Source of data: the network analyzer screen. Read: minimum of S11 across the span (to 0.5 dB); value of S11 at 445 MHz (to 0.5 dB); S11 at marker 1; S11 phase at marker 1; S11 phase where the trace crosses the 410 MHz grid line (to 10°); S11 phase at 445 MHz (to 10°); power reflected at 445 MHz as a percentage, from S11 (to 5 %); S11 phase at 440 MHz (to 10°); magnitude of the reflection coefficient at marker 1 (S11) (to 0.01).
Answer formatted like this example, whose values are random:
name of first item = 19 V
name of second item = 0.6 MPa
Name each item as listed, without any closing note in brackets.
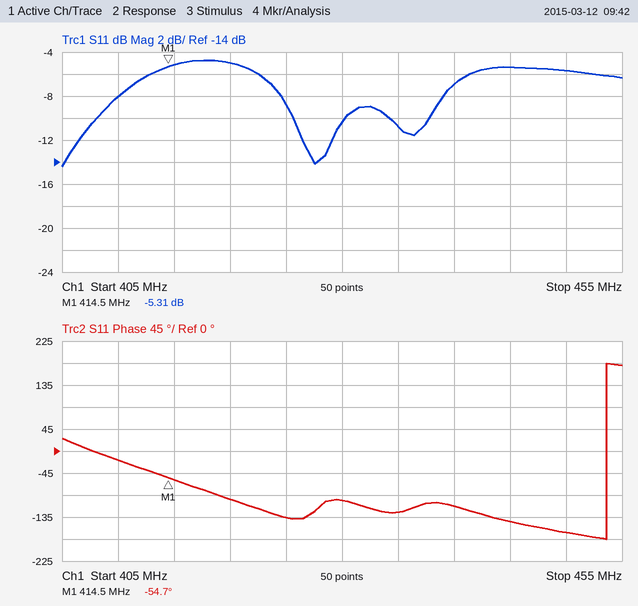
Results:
minimum of S11 across the span = -14.5 dB
value of S11 at 445 MHz = -5.5 dB
S11 at marker 1 = -5.31 dB
S11 phase at marker 1 = -54.7°
S11 phase where the trace crosses the 410 MHz grid line = -20°
S11 phase at 445 MHz = -140°
power reflected at 445 MHz as a percentage, from S11 = 30 %
S11 phase at 440 MHz = -110°
magnitude of the reflection coefficient at marker 1 (S11) = 0.54
